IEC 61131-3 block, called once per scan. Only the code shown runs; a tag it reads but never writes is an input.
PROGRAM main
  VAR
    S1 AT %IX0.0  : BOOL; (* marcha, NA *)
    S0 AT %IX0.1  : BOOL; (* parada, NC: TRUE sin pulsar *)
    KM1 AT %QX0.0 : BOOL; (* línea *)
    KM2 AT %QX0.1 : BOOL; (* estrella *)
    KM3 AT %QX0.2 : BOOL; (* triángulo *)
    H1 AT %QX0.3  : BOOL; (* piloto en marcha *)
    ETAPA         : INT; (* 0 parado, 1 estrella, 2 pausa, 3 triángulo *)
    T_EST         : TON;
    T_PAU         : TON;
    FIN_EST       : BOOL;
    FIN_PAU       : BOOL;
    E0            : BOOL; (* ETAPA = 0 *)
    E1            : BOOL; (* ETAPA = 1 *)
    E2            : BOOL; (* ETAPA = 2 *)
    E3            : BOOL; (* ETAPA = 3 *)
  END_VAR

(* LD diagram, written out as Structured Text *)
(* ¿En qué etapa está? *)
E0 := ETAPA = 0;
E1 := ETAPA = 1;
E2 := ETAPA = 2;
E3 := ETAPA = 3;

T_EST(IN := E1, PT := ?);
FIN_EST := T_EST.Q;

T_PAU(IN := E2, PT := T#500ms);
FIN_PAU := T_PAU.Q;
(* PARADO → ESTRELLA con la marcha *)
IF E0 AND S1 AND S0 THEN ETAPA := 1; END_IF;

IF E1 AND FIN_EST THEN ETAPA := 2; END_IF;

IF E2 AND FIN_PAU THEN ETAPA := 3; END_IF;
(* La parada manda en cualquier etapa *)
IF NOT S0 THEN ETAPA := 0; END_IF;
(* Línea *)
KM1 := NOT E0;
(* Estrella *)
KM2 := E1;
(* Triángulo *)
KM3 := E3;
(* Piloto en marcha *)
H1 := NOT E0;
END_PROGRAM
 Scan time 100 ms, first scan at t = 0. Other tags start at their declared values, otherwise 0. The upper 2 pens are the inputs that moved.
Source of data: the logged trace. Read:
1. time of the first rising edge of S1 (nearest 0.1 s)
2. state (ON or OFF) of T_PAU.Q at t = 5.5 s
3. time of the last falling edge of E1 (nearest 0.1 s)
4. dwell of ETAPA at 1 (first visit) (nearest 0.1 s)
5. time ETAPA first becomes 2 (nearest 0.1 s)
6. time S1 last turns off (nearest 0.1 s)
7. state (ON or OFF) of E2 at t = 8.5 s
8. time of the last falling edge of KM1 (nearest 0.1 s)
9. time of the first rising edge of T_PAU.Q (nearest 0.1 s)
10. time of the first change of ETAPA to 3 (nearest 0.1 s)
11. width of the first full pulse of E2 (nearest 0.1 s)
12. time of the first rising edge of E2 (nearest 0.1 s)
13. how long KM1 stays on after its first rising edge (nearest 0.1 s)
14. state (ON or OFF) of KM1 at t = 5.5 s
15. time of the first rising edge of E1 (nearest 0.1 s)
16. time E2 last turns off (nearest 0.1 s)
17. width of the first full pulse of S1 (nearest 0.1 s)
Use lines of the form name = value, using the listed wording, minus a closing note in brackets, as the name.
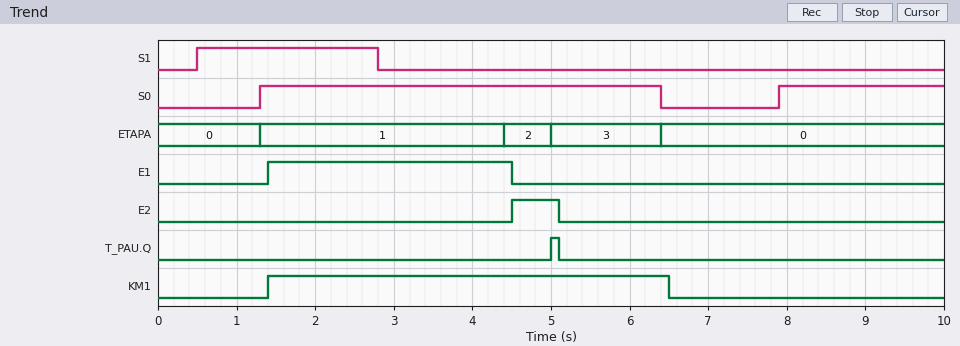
time of the first rising edge of S1 = 0.5 s
state (ON or OFF) of T_PAU.Q at t = 5.5 s = OFF
time of the last falling edge of E1 = 4.5 s
dwell of ETAPA at 1 (first visit) = 3.1 s
time ETAPA first becomes 2 = 4.4 s
time S1 last turns off = 2.8 s
state (ON or OFF) of E2 at t = 8.5 s = OFF
time of the last falling edge of KM1 = 6.5 s
time of the first rising edge of T_PAU.Q = 5.0 s
time of the first change of ETAPA to 3 = 5.0 s
width of the first full pulse of E2 = 0.6 s
time of the first rising edge of E2 = 4.5 s
how long KM1 stays on after its first rising edge = 5.1 s
state (ON or OFF) of KM1 at t = 5.5 s = ON
time of the first rising edge of E1 = 1.4 s
time E2 last turns off = 5.1 s
width of the first full pulse of S1 = 2.3 s
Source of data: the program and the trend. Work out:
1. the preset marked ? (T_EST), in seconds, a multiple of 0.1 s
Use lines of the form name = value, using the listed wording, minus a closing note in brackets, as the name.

the preset marked ? (T_EST), in seconds, a multiple of 0.1 s = 3.0 s
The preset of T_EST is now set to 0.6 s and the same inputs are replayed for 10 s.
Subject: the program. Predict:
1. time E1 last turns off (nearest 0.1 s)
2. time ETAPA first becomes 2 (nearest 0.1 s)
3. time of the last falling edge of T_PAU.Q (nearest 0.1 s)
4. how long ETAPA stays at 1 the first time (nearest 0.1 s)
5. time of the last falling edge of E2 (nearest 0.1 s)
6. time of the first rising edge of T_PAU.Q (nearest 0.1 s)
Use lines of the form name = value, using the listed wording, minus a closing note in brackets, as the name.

time E1 last turns off = 2.1 s
time ETAPA first becomes 2 = 2.0 s
time of the last falling edge of T_PAU.Q = 2.7 s
how long ETAPA stays at 1 the first time = 0.7 s
time of the last falling edge of E2 = 2.7 s
time of the first rising edge of T_PAU.Q = 2.6 s
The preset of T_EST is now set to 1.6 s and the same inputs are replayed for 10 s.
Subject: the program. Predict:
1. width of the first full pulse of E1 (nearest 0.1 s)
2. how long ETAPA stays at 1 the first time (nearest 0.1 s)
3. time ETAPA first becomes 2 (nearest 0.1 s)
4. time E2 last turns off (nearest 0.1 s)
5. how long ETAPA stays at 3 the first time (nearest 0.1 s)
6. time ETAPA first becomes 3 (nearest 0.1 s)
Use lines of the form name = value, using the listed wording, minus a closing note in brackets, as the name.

width of the first full pulse of E1 = 1.7 s
how long ETAPA stays at 1 the first time = 1.7 s
time ETAPA first becomes 2 = 3.0 s
time E2 last turns off = 3.7 s
how long ETAPA stays at 3 the first time = 2.8 s
time ETAPA first becomes 3 = 3.6 s
